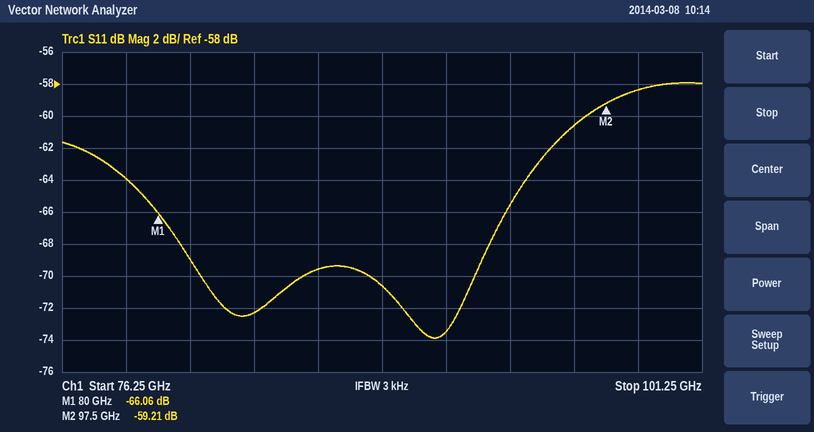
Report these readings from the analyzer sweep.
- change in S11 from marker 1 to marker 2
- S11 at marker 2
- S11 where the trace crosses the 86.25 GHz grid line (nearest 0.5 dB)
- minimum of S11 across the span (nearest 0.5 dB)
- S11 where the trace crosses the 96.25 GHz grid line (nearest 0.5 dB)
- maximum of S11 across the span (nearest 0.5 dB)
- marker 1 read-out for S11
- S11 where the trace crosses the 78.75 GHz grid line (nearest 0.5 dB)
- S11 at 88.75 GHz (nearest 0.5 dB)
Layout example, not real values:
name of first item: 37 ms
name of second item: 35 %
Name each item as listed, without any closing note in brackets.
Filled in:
change in S11 from marker 1 to marker 2: 6.85 dB
S11 at marker 2: -59.21 dB
S11 where the trace crosses the 86.25 GHz grid line: -69.5 dB
minimum of S11 across the span: -74.0 dB
S11 where the trace crosses the 96.25 GHz grid line: -60.5 dB
maximum of S11 across the span: -58.0 dB
marker 1 read-out for S11: -66.06 dB
S11 where the trace crosses the 78.75 GHz grid line: -64.0 dB
S11 at 88.75 GHz: -70.5 dB
